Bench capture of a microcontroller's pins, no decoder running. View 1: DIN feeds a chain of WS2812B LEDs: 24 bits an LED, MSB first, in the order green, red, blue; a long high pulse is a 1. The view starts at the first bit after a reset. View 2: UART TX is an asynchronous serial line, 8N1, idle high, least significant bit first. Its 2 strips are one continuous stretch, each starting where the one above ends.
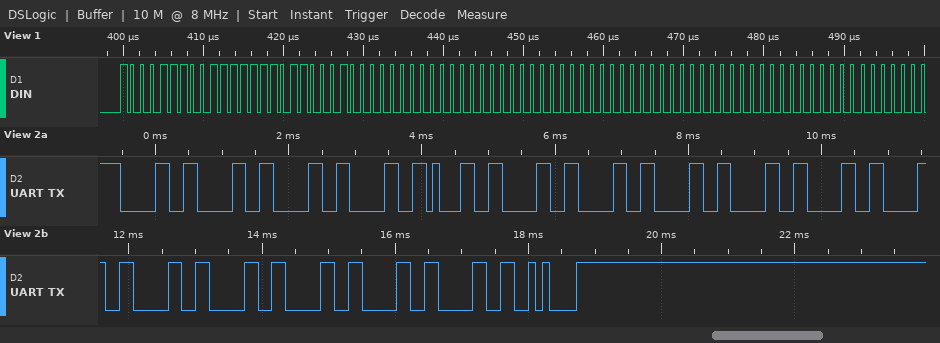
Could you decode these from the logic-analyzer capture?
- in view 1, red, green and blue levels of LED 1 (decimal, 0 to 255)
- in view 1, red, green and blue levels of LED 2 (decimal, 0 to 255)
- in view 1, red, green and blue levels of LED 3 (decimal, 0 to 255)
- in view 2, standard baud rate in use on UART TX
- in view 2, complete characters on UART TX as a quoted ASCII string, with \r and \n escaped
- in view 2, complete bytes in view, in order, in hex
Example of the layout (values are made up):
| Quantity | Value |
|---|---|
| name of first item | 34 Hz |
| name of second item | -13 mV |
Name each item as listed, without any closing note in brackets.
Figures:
| Quantity | Value |
|---|---|
| in view 1, red, green and blue levels of LED 1 | 127, 142, 98 |
| in view 1, red, green and blue levels of LED 2 | 0, 0, 0 |
| in view 1, red, green and blue levels of LED 3 | 0, 0, 0 |
| in view 2, standard baud rate in use on UART TX | 9600 baud |
| in view 2, complete characters on UART TX as a quoted ASCII string, with \r and \n escaped | "0000100000000000\n" |
| in view 2, complete bytes in view, in order, in hex | 30 30 30 30 31 30 30 30 30 30 30 30 30 30 30 30 0A |
